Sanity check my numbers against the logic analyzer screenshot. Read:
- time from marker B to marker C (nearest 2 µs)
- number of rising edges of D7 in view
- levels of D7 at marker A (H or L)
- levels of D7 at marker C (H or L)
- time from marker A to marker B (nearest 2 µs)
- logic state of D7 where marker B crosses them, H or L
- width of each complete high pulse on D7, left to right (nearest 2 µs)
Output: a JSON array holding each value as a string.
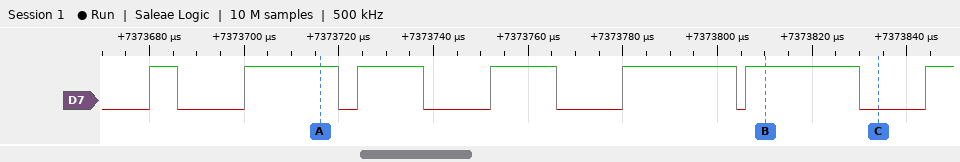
["24 µs", "7", "D7=H", "D7=L", "94 µs", "D7=H", "6 µs, 20 µs, 14 µs, 14 µs, 24 µs, 24 µs"]
